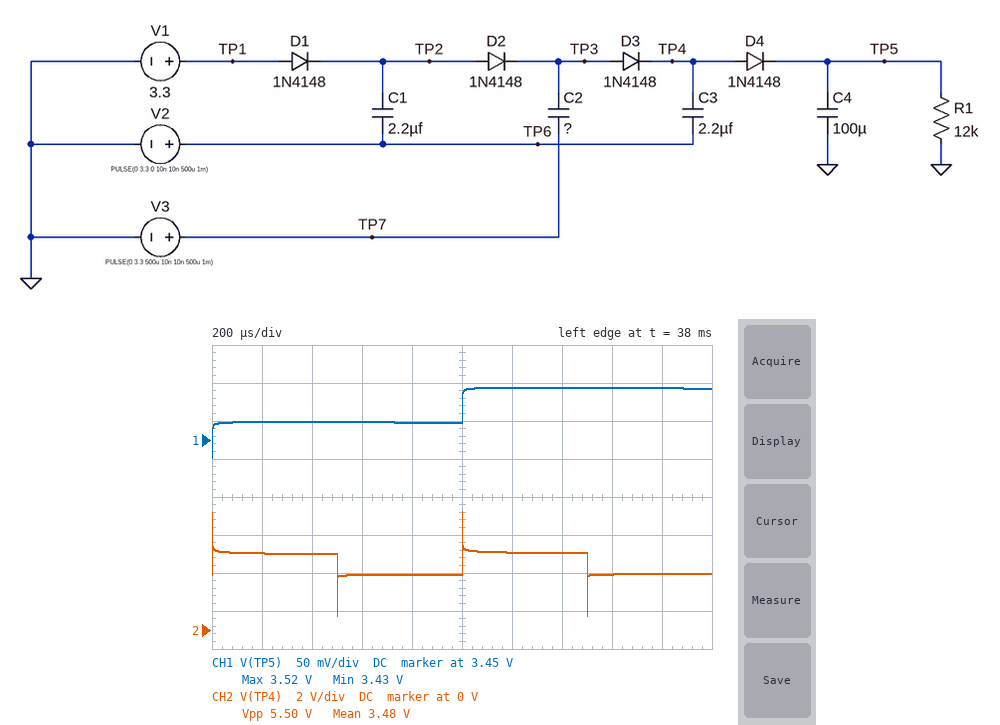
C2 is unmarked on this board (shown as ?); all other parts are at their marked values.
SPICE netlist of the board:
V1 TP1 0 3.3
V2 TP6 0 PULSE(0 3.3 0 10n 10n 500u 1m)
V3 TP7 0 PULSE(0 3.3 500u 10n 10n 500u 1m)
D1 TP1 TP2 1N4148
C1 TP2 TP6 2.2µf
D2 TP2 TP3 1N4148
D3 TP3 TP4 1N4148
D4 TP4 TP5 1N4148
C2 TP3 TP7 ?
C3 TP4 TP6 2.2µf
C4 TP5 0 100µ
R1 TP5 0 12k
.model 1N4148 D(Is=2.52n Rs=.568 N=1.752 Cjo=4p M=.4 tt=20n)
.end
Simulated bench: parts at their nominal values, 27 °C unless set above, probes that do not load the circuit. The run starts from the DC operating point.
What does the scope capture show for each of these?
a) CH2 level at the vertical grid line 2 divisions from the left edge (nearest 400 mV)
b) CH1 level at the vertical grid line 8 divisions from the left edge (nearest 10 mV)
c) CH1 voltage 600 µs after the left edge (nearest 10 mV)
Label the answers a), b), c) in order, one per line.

a) 4.0 V
b) 3.52 V
c) 3.47 V
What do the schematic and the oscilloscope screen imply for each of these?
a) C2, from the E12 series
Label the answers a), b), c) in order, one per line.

a) 1.5 µF
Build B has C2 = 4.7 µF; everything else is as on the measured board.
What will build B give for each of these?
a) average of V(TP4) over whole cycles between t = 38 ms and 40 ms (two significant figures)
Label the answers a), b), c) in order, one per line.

a) 4.6 V
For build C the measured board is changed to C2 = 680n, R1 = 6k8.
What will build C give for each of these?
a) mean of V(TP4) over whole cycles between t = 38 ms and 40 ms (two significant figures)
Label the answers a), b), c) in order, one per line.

a) 2.9 V
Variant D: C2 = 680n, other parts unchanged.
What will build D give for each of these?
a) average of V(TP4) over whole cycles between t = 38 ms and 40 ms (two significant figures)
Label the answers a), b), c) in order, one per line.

a) 2.9 V
